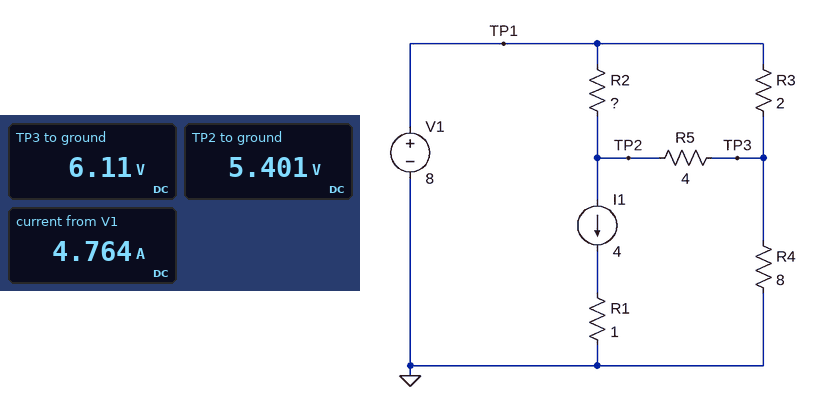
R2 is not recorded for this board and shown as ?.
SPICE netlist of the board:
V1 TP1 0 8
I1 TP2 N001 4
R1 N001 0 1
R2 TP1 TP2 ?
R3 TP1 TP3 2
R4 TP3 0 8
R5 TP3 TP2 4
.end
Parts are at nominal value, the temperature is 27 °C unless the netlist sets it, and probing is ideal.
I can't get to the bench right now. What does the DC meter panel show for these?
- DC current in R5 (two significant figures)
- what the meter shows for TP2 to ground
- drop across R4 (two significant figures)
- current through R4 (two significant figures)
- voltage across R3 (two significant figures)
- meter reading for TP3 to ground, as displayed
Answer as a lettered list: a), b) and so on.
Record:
a) 180 mA
b) 5.401 V
c) 6.1 V
d) 760 mA
e) 1.9 V
f) 6.11 V
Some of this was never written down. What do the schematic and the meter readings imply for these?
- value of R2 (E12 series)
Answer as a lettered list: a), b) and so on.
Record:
a) 0.68 Ω
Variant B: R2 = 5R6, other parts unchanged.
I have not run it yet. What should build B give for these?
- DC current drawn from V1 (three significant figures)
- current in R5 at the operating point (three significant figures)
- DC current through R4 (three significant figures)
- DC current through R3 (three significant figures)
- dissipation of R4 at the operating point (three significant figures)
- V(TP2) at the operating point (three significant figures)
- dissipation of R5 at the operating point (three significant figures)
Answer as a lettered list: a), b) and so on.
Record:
a) 4.43 A
b) 1.86 A
c) 429 mA
d) 2.29 A
e) 1.47 W
f) -4.00 V
g) 13.8 W
